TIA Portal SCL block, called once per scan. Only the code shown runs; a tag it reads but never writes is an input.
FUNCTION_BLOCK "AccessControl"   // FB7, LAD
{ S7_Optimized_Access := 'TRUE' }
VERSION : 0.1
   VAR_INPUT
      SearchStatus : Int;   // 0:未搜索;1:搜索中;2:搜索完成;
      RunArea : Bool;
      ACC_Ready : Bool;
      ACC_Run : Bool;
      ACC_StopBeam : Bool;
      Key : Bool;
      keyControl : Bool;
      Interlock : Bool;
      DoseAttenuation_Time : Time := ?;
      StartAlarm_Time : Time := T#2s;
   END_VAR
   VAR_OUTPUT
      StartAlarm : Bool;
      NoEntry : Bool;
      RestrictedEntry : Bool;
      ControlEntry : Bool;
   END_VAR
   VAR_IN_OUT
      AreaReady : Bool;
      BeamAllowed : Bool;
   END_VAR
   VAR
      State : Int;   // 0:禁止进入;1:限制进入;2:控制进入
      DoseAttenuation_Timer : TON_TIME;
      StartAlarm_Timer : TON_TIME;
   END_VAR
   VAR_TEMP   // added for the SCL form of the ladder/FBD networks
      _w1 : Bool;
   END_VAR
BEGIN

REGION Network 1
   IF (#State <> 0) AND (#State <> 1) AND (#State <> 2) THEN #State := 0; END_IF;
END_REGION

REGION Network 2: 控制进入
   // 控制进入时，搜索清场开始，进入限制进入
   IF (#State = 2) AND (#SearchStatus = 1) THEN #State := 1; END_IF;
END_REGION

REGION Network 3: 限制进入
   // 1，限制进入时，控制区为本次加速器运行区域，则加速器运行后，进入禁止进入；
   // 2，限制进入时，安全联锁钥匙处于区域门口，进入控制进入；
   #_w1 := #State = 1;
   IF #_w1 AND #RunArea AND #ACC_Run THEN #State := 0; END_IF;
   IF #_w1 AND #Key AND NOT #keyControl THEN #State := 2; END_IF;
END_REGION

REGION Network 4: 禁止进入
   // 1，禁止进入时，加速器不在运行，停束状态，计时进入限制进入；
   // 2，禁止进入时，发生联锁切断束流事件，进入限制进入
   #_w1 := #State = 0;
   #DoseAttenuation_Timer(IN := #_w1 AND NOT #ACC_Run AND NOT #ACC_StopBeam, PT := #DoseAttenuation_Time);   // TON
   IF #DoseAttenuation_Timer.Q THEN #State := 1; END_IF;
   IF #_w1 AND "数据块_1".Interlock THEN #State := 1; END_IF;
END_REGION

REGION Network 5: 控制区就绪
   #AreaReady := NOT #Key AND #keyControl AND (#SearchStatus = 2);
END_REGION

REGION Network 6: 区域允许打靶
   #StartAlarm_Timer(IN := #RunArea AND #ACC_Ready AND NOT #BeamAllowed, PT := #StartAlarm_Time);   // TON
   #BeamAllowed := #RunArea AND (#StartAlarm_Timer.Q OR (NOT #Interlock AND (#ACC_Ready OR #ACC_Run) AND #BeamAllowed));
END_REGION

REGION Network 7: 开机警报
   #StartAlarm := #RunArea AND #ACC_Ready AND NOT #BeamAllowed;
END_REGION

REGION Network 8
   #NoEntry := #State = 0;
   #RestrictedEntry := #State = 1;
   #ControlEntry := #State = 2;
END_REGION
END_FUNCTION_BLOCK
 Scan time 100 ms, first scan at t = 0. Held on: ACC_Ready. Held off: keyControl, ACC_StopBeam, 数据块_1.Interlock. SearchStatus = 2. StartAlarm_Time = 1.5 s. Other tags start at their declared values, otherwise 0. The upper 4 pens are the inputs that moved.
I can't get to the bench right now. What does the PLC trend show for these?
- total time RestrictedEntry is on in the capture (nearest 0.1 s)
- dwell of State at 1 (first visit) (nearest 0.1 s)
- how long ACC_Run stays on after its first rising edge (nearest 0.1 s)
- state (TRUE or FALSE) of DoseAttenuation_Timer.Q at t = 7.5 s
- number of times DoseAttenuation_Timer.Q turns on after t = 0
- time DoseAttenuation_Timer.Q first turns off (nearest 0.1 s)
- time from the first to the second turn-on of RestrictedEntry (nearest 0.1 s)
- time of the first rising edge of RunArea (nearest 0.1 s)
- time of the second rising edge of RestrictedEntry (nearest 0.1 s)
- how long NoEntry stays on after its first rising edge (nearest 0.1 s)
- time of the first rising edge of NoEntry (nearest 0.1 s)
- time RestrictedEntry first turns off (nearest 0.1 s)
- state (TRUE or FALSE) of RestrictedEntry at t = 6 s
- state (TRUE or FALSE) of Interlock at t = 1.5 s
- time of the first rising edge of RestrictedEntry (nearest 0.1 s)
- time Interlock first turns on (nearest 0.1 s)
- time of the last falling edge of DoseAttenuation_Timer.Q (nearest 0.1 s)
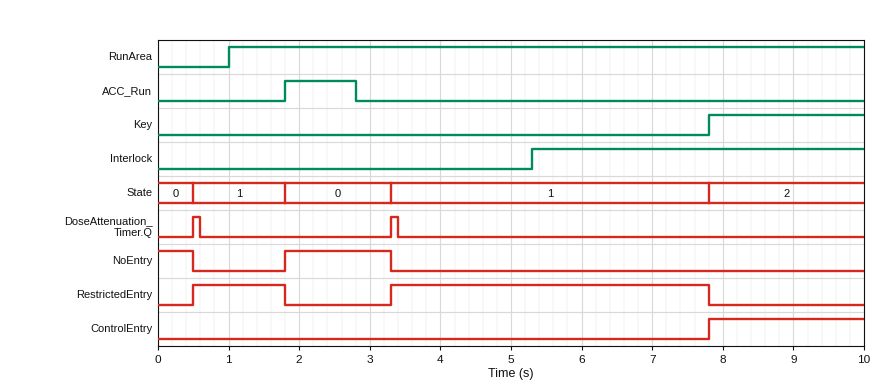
5.8 s
1.3 s
1.0 s
FALSE
2
0.6 s
2.8 s
1.0 s
3.3 s
1.5 s
1.8 s
1.8 s
TRUE
FALSE
0.5 s
5.3 s
3.4 s
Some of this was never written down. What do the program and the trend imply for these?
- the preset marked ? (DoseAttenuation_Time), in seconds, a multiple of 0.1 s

0.5 s
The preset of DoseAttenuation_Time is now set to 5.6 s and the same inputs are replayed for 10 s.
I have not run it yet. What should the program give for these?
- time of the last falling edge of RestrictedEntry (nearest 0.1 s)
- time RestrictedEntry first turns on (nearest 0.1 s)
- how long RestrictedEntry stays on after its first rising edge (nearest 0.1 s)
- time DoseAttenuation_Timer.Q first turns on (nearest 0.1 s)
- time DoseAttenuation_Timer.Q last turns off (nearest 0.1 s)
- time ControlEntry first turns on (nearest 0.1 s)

8.5 s
8.4 s
0.1 s
8.4 s
8.5 s
8.5 s
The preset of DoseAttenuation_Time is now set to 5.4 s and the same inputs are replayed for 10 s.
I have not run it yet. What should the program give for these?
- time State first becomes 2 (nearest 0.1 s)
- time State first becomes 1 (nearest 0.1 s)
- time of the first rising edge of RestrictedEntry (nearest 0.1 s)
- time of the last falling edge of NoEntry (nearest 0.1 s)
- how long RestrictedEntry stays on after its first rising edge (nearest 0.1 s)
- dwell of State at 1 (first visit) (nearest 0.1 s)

8.3 s
8.2 s
8.2 s
8.2 s
0.1 s
0.1 s
